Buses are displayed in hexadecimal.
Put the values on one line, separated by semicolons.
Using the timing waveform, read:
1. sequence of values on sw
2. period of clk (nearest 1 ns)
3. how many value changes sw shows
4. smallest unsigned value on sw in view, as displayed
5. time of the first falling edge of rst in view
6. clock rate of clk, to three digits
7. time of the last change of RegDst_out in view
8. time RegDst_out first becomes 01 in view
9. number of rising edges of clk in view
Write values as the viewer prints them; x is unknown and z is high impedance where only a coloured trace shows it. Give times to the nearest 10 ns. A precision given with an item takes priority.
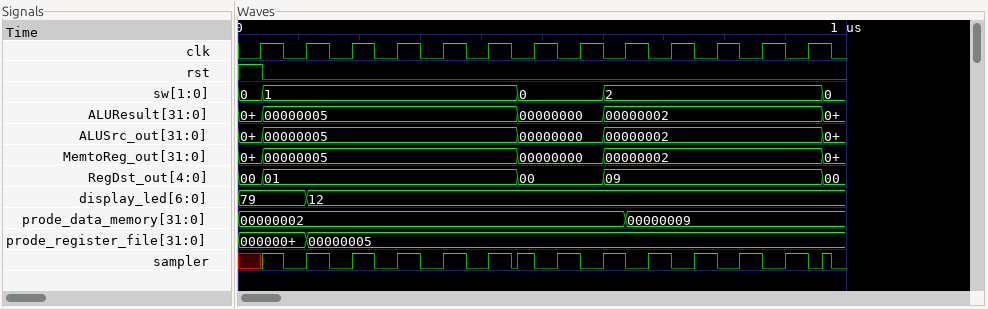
0, 1, 0, 2, 0; 75 ns; 4; 0; 40 ns; 13.3 MHz; 960 ns; 40 ns; 13
